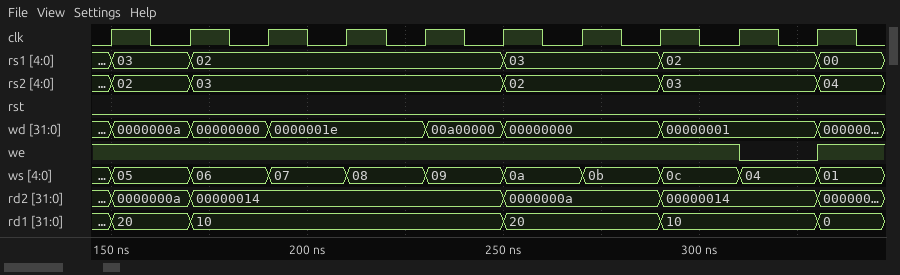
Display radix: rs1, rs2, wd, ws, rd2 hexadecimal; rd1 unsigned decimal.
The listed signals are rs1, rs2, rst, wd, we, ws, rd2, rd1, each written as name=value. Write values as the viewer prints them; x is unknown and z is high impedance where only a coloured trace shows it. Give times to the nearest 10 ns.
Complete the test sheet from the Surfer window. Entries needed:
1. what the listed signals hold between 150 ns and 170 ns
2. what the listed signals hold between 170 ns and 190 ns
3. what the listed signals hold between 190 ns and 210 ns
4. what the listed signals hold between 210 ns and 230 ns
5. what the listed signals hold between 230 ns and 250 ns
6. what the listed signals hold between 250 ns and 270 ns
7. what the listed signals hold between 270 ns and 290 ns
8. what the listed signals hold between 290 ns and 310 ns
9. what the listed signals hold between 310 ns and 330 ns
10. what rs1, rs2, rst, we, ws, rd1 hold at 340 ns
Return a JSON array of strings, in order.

["rs1=03, rs2=02, rst=0, wd=0000000a, we=1, ws=05, rd2=0000000a, rd1=20", "rs1=02, rs2=03, rst=0, wd=00000000, we=1, ws=06, rd2=00000014, rd1=10", "rs1=02, rs2=03, rst=0, wd=0000001e, we=1, ws=07, rd2=00000014, rd1=10", "rs1=02, rs2=03, rst=0, wd=0000001e, we=1, ws=08, rd2=00000014, rd1=10", "rs1=02, rs2=03, rst=0, wd=00a00000, we=1, ws=09, rd2=00000014, rd1=10", "rs1=03, rs2=02, rst=0, wd=00000000, we=1, ws=0a, rd2=0000000a, rd1=20", "rs1=03, rs2=02, rst=0, wd=00000000, we=1, ws=0b, rd2=0000000a, rd1=20", "rs1=02, rs2=03, rst=0, wd=00000001, we=1, ws=0c, rd2=00000014, rd1=10", "rs1=02, rs2=03, rst=0, wd=00000001, we=0, ws=04, rd2=00000014, rd1=10", "rs1=00, rs2=04, rst=0, we=1, ws=01, rd1=0"]
